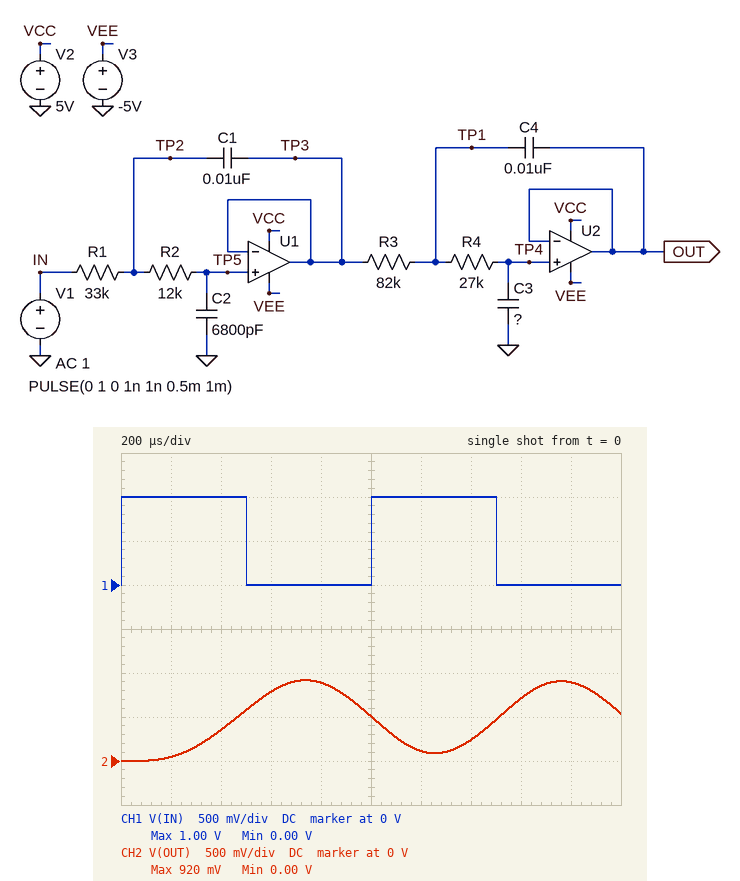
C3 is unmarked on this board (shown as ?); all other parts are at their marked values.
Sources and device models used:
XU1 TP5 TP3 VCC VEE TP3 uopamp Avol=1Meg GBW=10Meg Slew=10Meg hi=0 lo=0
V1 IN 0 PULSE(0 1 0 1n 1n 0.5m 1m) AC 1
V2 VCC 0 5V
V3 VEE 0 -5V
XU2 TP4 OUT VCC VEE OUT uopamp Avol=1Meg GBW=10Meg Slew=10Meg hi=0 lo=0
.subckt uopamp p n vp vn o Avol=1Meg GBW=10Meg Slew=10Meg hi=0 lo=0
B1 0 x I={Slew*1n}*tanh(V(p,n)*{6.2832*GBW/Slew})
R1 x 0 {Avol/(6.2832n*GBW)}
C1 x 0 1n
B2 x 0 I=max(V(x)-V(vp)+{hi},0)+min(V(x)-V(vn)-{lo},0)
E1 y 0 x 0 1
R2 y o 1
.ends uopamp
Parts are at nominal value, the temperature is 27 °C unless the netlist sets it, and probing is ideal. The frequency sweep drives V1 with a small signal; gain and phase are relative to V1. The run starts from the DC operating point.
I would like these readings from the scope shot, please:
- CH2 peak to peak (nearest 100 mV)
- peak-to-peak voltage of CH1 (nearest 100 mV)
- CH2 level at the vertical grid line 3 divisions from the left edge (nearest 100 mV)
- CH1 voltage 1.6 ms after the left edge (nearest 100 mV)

900 mV
1.0 V
800 mV
0 V
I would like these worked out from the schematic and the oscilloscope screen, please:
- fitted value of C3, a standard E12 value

1.2 nF
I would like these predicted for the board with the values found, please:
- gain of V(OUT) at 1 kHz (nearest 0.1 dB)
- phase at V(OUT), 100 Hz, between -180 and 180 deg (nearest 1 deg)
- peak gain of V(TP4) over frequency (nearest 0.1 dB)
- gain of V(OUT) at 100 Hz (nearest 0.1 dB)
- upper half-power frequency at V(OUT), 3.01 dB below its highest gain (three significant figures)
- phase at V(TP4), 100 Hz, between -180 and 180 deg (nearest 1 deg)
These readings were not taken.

-4.0 dB
-16 deg
0 dB
0 dB
944 Hz
-16 deg
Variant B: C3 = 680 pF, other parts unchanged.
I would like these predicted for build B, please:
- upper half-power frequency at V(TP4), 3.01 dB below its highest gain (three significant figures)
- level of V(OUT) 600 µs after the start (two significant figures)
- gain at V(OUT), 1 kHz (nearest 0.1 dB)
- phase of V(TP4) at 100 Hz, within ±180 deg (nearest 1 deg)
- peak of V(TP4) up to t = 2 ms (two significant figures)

1.23 kHz
970 mV
-1.5 dB
-14 deg
1.0 V
